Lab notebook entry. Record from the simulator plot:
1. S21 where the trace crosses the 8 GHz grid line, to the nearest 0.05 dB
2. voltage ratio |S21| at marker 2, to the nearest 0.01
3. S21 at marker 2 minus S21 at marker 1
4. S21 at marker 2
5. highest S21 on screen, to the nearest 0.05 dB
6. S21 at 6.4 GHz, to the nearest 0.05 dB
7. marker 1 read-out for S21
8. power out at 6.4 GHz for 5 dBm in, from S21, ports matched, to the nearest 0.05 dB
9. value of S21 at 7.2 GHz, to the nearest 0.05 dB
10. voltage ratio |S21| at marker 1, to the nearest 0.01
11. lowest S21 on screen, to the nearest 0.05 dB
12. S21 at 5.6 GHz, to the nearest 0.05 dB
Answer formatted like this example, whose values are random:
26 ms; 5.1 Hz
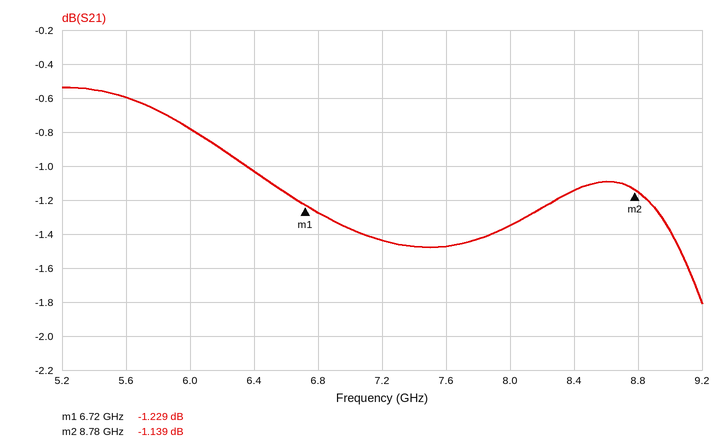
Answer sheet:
-1.35 dB; 0.88; 0.090 dB; -1.139 dB; -0.55 dB; -1.05 dB; -1.229 dB; 3.95 dBm; -1.45 dB; 0.87; -1.80 dB; -0.60 dB
